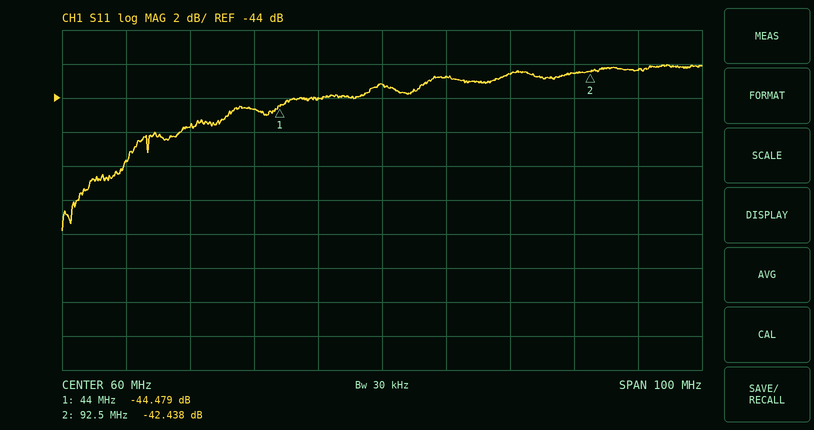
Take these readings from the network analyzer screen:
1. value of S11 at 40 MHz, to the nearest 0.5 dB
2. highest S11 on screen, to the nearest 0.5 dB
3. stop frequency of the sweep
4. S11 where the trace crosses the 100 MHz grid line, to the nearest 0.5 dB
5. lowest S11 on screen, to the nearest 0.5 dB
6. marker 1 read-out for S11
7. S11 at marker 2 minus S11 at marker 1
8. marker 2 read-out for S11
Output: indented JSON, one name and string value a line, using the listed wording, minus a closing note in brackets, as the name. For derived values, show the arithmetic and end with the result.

{
  "value of S11 at 40 MHz, to the nearest 0.5 dB": "-44.5 dB",
  "highest S11 on screen, to the nearest 0.5 dB": "-42.0 dB",
  "stop frequency of the sweep": "110 MHz",
  "S11 where the trace crosses the 100 MHz grid line, to the nearest 0.5 dB": "-42.5 dB",
  "lowest S11 on screen, to the nearest 0.5 dB": "-52.0 dB",
  "marker 1 read-out for S11": "-44.479 dB",
  "S11 at marker 2 minus S11 at marker 1": "-42.438 − (-44.479) = 2.041 dB",
  "marker 2 read-out for S11": "-42.438 dB"
}
